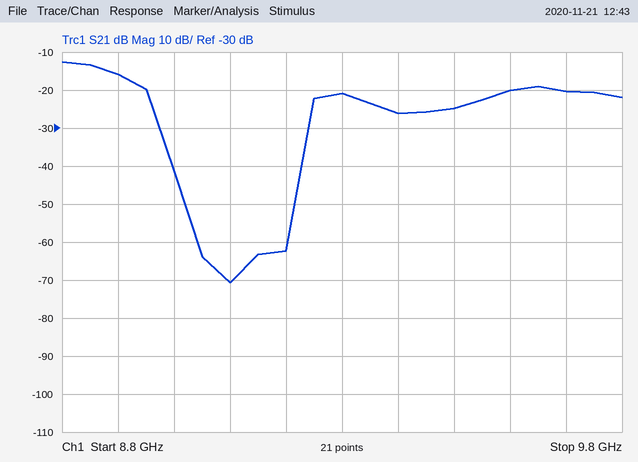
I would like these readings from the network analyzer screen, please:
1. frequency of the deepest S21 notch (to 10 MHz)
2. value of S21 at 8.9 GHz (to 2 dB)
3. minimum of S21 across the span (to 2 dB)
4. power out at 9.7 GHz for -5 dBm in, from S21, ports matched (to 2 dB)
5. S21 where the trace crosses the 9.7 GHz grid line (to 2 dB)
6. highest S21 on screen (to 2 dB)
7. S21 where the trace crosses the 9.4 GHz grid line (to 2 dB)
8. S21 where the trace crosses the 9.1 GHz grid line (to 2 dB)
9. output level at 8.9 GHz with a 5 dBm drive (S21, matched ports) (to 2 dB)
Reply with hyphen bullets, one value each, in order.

- 9.10 GHz
- -16 dB
- -70 dB
- -26 dBm
- -20 dB
- -12 dB
- -26 dB
- -70 dB
- -10 dBm
